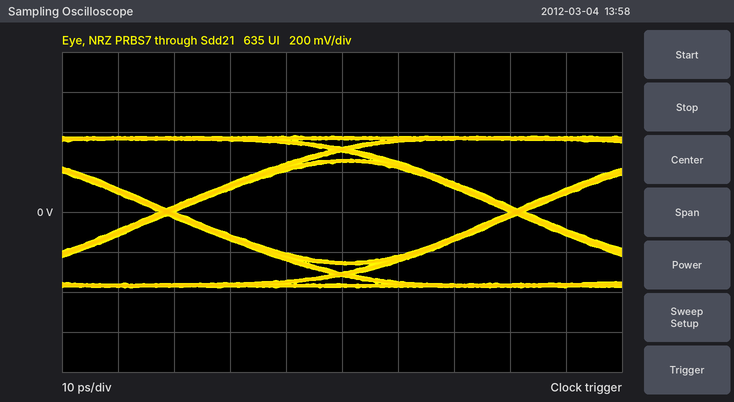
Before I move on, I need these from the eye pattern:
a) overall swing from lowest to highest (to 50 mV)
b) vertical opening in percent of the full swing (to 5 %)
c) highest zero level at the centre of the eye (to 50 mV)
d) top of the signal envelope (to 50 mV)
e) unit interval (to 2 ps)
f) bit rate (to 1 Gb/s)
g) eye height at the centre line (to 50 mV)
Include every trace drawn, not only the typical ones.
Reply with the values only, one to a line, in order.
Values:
750 mV
65 %
-250 mV
400 mV
62 ps
16 Gb/s
500 mV
